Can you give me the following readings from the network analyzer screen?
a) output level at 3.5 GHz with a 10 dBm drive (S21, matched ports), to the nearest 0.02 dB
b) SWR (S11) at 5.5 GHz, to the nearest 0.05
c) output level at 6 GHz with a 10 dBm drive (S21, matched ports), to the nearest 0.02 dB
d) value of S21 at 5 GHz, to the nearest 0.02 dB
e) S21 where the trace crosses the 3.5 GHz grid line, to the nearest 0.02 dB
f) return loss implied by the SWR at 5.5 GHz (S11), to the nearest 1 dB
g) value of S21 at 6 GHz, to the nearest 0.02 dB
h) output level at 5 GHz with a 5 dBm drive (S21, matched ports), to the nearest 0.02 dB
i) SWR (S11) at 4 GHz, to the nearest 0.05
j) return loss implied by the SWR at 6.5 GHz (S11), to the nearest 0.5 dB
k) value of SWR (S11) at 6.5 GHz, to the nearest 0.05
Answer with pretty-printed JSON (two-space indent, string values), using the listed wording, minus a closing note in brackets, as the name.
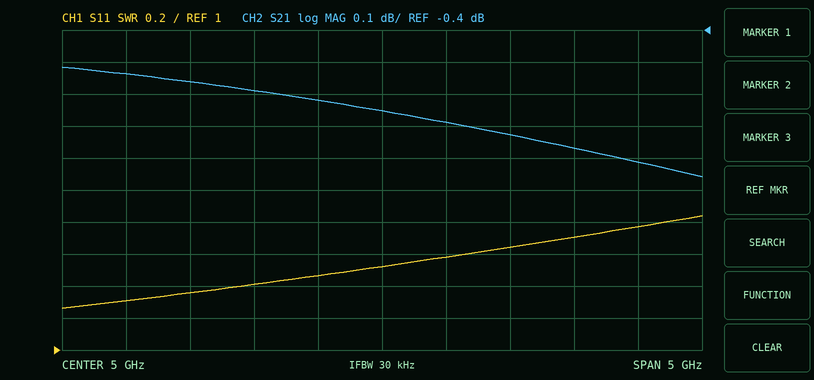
{
  "output level at 3.5 GHz with a 10 dBm drive (S21, matched ports), to the nearest 0.02 dB": "9.44 dBm",
  "SWR (S11) at 5.5 GHz, to the nearest 0.05": "1.60",
  "output level at 6 GHz with a 10 dBm drive (S21, matched ports), to the nearest 0.02 dB": "9.28 dBm",
  "value of S21 at 5 GHz, to the nearest 0.02 dB": "-0.66 dB",
  "S21 where the trace crosses the 3.5 GHz grid line, to the nearest 0.02 dB": "-0.56 dB",
  "return loss implied by the SWR at 5.5 GHz (S11), to the nearest 1 dB": "13 dB",
  "value of S21 at 6 GHz, to the nearest 0.02 dB": "-0.72 dB",
  "output level at 5 GHz with a 5 dBm drive (S21, matched ports), to the nearest 0.02 dB": "4.34 dBm",
  "SWR (S11) at 4 GHz, to the nearest 0.05": "1.40",
  "return loss implied by the SWR at 6.5 GHz (S11), to the nearest 0.5 dB": "11.5 dB",
  "value of SWR (S11) at 6.5 GHz, to the nearest 0.05": "1.70"
}
